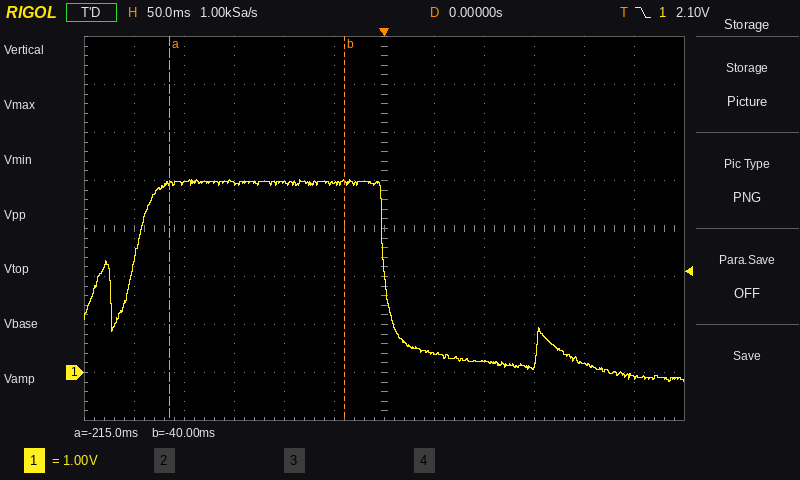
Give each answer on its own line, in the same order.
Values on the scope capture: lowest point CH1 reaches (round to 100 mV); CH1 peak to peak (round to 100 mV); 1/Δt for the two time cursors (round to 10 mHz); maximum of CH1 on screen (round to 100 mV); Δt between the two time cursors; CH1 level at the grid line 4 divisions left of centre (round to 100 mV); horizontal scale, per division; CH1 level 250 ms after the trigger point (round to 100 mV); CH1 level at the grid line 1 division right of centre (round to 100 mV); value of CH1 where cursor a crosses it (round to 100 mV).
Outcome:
-200 mV
4.2 V
5.71 Hz
4.0 V
175 ms
3.9 V
50 ms
-100 mV
400 mV
3.9 V
